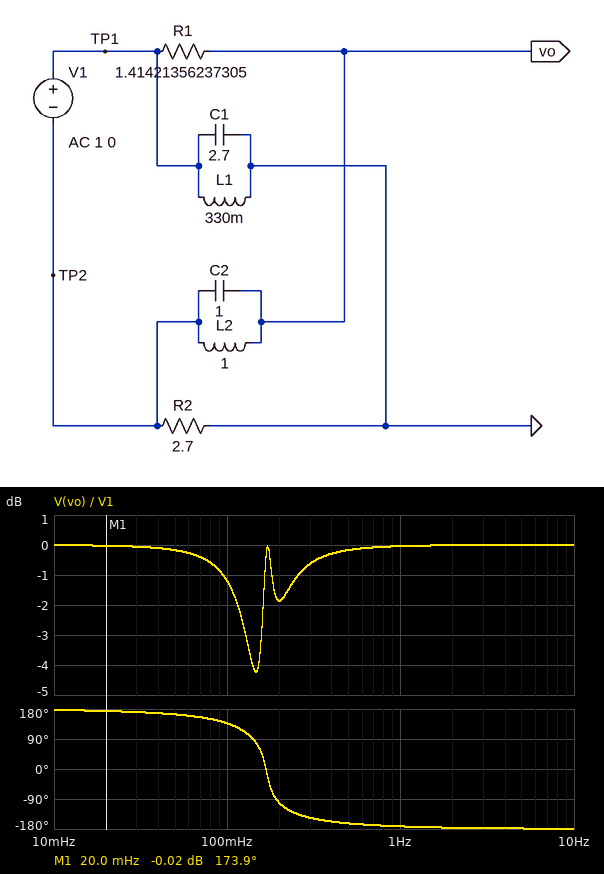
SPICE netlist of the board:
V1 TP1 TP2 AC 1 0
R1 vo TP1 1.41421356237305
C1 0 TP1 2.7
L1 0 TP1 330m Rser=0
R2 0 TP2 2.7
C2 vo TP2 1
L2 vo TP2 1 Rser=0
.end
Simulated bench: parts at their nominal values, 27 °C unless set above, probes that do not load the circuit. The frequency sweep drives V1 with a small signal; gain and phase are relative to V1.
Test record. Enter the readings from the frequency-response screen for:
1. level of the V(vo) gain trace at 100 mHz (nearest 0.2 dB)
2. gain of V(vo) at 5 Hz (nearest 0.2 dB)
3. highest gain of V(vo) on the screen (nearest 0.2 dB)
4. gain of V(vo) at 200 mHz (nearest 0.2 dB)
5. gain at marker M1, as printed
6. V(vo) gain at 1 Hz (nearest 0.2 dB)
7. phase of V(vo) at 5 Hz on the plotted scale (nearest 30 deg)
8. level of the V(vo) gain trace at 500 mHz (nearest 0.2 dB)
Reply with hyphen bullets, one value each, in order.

- -1.2 dB
- 0 dB
- 0 dB
- -1.8 dB
- -0.02 dB
- 0 dB
- -180 deg
- -0.2 dB
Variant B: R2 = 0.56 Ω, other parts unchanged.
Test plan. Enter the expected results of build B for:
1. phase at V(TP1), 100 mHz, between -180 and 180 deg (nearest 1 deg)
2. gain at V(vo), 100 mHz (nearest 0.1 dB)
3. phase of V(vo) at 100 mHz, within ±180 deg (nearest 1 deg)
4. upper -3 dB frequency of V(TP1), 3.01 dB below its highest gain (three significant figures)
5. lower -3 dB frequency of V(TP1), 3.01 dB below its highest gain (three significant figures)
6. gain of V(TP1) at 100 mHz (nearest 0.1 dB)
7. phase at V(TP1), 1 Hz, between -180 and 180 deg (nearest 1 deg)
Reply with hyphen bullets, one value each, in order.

- 60 deg
- -0.1 dB
- 114 deg
- 229 mHz
- 124 mHz
- -6.1 dB
- -84 deg
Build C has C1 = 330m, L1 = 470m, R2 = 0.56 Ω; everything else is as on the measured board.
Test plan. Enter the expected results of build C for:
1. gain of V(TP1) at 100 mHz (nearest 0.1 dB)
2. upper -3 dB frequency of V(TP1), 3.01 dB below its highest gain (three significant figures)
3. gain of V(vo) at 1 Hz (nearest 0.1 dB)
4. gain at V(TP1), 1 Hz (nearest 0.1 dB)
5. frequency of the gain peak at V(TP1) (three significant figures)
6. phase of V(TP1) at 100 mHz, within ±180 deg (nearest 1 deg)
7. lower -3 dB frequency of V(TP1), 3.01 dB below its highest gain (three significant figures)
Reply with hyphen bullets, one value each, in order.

- -6.2 dB
- 1.02 Hz
- -2.2 dB
- -2.9 dB
- 404 mHz
- 61 deg
- 160 mHz
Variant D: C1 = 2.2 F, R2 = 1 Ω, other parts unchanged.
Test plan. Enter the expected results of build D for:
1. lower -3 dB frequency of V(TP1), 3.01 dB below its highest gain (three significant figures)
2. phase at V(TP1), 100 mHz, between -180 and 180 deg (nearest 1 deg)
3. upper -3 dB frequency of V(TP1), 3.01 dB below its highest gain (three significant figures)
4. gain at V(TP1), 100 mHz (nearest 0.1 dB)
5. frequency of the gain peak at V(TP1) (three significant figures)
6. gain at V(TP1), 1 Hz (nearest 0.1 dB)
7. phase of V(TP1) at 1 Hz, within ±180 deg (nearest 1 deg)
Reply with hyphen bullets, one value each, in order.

- 154 mHz
- 74 deg
- 226 mHz
- -11.1 dB
- 187 mHz
- -22.5 dB
- -86 deg
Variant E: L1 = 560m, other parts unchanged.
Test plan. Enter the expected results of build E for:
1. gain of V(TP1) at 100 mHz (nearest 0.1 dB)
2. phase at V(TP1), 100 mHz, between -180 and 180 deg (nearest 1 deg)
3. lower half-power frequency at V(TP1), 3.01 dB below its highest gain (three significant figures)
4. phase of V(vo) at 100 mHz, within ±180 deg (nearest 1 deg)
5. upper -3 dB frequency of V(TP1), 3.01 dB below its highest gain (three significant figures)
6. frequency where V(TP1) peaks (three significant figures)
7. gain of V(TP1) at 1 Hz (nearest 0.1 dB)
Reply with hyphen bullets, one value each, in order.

- -10.2 dB
- 72 deg
- 119 mHz
- 126 deg
- 141 mHz
- 129 mHz
- -33.1 dB
